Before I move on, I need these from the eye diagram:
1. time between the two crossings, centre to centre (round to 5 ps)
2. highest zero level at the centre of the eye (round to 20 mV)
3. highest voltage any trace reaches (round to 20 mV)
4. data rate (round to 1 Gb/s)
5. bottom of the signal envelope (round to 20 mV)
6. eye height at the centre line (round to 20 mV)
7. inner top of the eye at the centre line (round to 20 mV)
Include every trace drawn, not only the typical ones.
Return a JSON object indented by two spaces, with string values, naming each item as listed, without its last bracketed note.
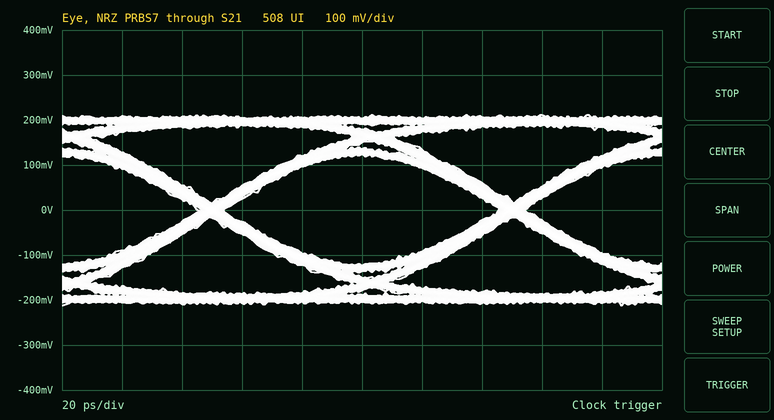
{
  "time between the two crossings, centre to centre": "100 ps",
  "highest zero level at the centre of the eye": "-120 mV",
  "highest voltage any trace reaches": "220 mV",
  "data rate": "10 Gb/s",
  "bottom of the signal envelope": "-220 mV",
  "eye height at the centre line": "240 mV",
  "inner top of the eye at the centre line": "120 mV"
}
